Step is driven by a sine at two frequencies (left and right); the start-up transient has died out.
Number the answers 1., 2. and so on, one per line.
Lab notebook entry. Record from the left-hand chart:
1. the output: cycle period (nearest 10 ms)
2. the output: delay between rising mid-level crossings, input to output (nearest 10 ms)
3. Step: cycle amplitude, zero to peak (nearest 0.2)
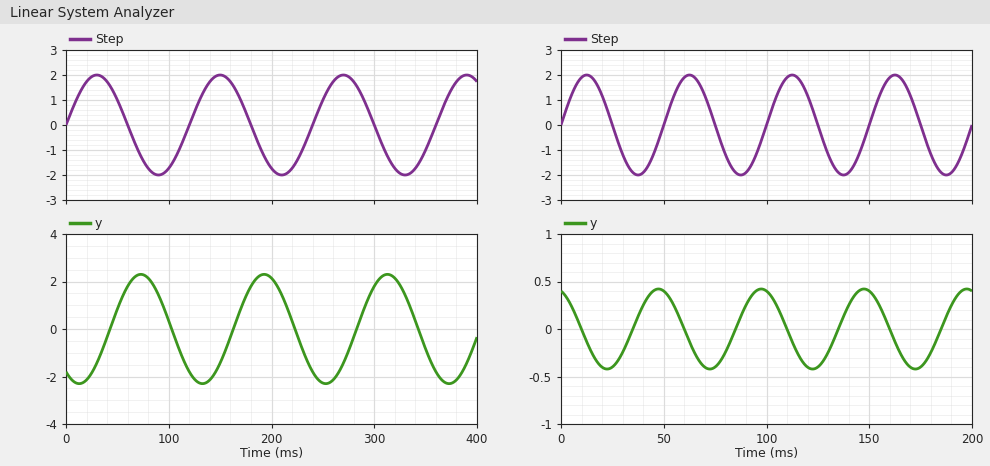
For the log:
1. 120 ms
2. 40 ms
3. 2.0
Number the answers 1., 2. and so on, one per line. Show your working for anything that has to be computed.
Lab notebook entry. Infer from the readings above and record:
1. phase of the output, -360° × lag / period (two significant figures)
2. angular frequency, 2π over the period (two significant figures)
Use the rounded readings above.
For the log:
1. -360 × 40 / 120 = -120°
2. 2π / 120 = 0.052 rad/ms
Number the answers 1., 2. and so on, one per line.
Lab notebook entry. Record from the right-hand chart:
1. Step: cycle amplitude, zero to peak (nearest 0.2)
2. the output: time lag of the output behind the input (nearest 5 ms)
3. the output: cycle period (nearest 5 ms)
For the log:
1. 2.0
2. 35 ms
3. 50 ms
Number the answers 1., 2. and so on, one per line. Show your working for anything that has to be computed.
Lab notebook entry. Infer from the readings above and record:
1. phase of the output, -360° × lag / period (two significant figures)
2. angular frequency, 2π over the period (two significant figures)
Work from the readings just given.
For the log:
1. -360 × 35 / 50 = -250°
2. 2π / 50 = 0.13 rad/ms
